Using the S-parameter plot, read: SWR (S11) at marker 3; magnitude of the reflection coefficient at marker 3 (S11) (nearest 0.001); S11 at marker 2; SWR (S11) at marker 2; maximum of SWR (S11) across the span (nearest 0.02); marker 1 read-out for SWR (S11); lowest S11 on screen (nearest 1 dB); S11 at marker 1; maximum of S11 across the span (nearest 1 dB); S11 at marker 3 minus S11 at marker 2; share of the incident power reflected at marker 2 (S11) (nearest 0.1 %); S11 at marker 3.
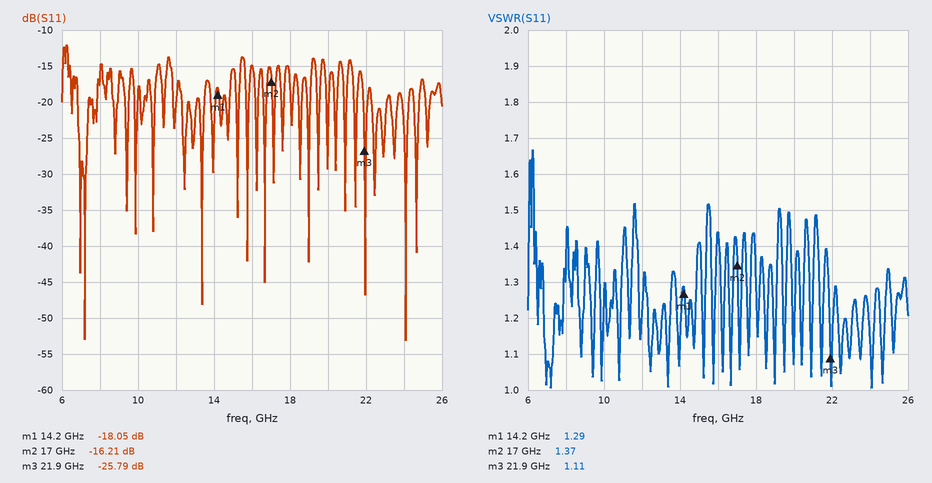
1.11
0.051
-16.21 dB
1.37
1.66
1.29
-53 dB
-18.05 dB
-12 dB
-9.58 dB
2.4 %
-25.79 dB
